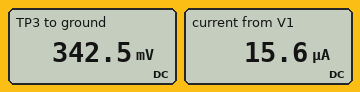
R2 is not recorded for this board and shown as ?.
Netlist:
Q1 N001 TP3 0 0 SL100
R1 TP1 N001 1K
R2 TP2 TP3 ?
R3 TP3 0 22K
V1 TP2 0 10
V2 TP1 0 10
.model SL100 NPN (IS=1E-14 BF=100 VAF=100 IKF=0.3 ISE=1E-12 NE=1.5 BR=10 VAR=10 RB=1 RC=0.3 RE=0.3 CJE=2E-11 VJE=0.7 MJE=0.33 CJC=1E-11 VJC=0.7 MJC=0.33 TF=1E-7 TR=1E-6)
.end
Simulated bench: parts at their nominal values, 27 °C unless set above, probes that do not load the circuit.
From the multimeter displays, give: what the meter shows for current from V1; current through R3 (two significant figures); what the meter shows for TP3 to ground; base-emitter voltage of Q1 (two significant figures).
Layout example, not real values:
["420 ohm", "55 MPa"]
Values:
["15.6 µA", "16 µA", "342.5 mV", "340 mV"]
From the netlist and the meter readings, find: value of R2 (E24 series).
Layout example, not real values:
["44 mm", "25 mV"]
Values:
["620 kΩ"]
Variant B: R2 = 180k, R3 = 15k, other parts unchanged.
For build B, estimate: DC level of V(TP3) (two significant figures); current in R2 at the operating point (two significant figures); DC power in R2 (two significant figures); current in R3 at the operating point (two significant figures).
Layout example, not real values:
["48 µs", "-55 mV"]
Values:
["620 mV", "52 µA", "490 µW", "41 µA"]
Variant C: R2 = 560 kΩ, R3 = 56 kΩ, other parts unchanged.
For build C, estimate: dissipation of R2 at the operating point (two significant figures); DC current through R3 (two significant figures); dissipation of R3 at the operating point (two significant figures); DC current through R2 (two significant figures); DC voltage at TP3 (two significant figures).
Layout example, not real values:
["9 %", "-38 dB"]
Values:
["160 µW", "11 µA", "6.4 µW", "17 µA", "600 mV"]
